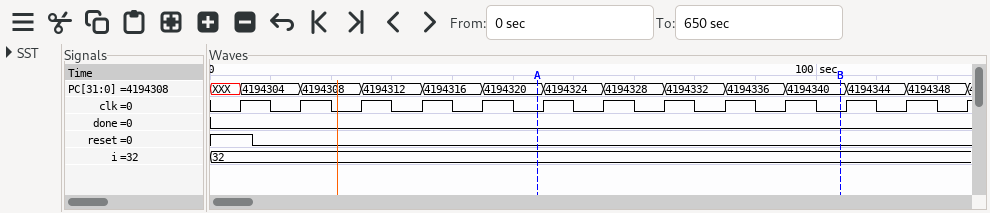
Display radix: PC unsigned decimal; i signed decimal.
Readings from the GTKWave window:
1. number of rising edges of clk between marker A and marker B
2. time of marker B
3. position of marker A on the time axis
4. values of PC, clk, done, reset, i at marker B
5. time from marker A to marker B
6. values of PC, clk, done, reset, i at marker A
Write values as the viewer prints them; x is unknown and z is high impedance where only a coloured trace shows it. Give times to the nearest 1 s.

5
104 s
54 s
PC=4194340, clk=0, done=0, reset=0, i=32
50 s
PC=4194320, clk=0, done=0, reset=0, i=32
